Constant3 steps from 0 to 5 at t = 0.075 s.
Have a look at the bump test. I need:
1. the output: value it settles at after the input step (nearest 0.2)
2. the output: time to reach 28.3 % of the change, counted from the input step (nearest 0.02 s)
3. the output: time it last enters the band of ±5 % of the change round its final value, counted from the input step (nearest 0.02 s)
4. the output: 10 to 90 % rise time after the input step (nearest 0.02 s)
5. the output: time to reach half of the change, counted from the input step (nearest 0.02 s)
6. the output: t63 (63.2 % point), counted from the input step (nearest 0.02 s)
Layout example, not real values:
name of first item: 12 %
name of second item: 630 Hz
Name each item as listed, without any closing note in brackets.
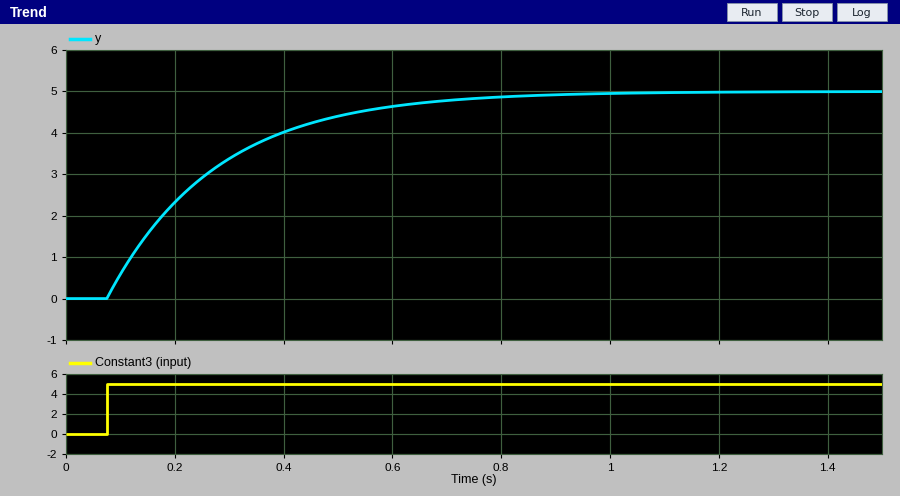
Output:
the output: value it settles at after the input step: 5.0
the output: time to reach 28.3 % of the change, counted from the input step: 0.06 s
the output: time it last enters the band of ±5 % of the change round its final value, counted from the input step: 0.60 s
the output: 10 to 90 % rise time after the input step: 0.44 s
the output: time to reach half of the change, counted from the input step: 0.14 s
the output: t63 (63.2 % point), counted from the input step: 0.20 s
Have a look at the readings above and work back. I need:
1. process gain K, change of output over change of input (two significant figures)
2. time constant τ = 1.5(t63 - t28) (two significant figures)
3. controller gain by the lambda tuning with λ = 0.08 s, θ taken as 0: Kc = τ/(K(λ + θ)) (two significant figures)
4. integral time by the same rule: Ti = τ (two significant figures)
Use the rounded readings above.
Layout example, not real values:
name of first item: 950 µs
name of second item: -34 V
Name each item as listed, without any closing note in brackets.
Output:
process gain K, change of output over change of input: 1.0
time constant τ = 1.5(t63 - t28): 0.21 s
controller gain by the lambda tuning with λ = 0.08 s, θ taken as 0: Kc = τ/(K(λ + θ)): 2.6
integral time by the same rule: Ti = τ: 0.21 s
